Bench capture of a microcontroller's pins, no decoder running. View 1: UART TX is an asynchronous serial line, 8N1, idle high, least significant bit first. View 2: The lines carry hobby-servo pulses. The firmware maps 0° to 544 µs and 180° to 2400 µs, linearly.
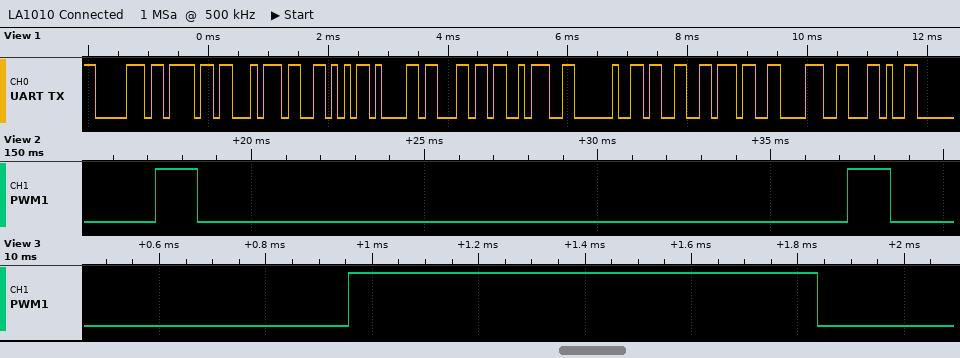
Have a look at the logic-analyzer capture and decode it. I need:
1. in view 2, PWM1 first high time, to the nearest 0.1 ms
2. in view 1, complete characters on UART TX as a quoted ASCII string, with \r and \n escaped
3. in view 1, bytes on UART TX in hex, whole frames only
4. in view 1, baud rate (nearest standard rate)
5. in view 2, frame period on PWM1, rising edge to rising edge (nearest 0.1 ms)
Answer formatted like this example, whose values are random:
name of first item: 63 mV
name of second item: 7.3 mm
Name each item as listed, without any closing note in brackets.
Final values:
in view 2, PWM1 first high time, to the nearest 0.1 ms: 1.2 ms
in view 1, complete characters on UART TX as a quoted ASCII string, with \r and \n escaped: "potVal: 378,"
in view 1, bytes on UART TX in hex, whole frames only: 70 6F 74 56 61 6C 3A 20 33 37 38 2C
in view 1, baud rate: 9600 baud
in view 2, frame period on PWM1, rising edge to rising edge: 20.0 ms
